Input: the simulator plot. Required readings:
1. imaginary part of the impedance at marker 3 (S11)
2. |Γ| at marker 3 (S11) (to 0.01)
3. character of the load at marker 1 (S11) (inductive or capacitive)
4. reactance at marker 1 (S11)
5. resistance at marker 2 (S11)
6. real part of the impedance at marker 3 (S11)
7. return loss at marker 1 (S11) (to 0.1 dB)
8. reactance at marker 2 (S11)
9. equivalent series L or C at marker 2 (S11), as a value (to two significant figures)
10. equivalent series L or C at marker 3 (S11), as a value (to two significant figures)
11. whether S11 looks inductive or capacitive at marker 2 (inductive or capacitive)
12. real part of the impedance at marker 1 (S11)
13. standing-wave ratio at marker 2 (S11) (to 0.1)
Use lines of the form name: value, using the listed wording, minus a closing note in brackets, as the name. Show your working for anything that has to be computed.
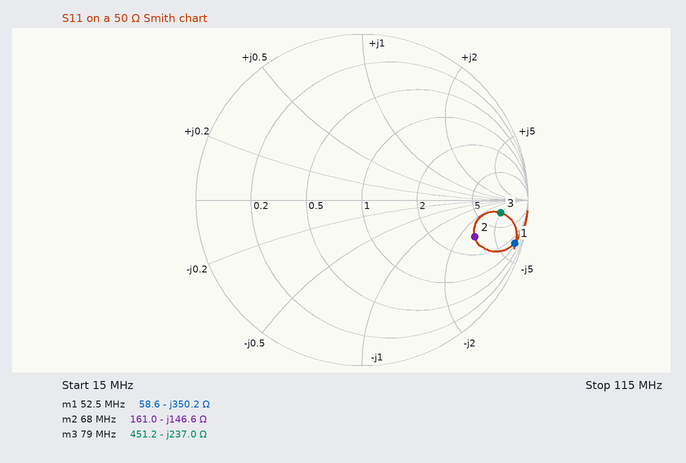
imaginary part of the impedance at marker 3: -237.0 Ω
|Γ| at marker 3 (S11): 0.84
character of the load at marker 1 (S11): capacitive
reactance at marker 1: -350.2 Ω
resistance at marker 2: 161.0 Ω
real part of the impedance at marker 3: 451.2 Ω
return loss at marker 1 (S11): 0.4 dB
reactance at marker 2: -146.6 Ω
equivalent series L or C at marker 2 (S11), as a value: C = 1/(2π × 68 MHz × 146.6 Ω) ≈ 16 pF
equivalent series L or C at marker 3 (S11), as a value: C = 1/(2π × 79 MHz × 237 Ω) ≈ 8.5 pF
whether S11 looks inductive or capacitive at marker 2: capacitive
real part of the impedance at marker 1: 58.6 Ω
standing-wave ratio at marker 2 (S11): 6.0
